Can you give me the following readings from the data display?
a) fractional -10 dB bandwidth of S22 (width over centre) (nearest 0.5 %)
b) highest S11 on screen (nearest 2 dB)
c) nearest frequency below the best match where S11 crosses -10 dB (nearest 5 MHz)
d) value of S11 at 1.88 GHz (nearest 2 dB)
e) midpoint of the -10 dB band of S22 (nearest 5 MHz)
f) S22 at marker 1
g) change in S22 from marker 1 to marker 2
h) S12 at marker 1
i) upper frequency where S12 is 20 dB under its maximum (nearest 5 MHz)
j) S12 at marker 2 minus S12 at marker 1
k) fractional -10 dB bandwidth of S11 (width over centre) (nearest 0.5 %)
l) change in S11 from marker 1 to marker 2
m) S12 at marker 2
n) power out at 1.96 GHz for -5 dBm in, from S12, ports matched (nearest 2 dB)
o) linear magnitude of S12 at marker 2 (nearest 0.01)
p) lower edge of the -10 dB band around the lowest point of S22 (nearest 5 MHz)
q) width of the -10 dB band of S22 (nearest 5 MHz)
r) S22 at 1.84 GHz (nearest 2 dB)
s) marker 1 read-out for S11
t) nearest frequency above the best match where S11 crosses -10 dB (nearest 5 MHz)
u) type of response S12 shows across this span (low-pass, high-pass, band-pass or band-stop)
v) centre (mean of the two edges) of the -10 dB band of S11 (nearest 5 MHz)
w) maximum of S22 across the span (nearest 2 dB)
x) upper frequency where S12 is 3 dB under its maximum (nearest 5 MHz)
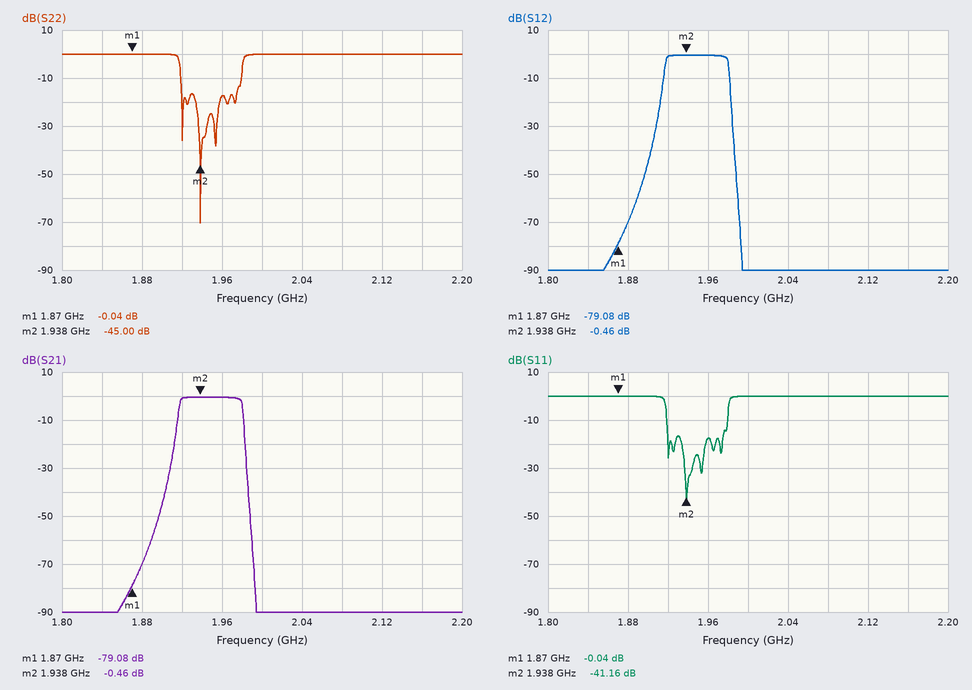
3.0 %
0 dB
1.920 GHz
0 dB
1.950 GHz
-0.04 dB
-44.96 dB
-79.08 dB
1.985 GHz
78.62 dB
3.0 %
-41.12 dB
-0.46 dB
-6 dBm
0.95
1.920 GHz
60 MHz
0 dB
-0.04 dB
1.980 GHz
band-pass
1.950 GHz
0 dB
1.980 GHz
